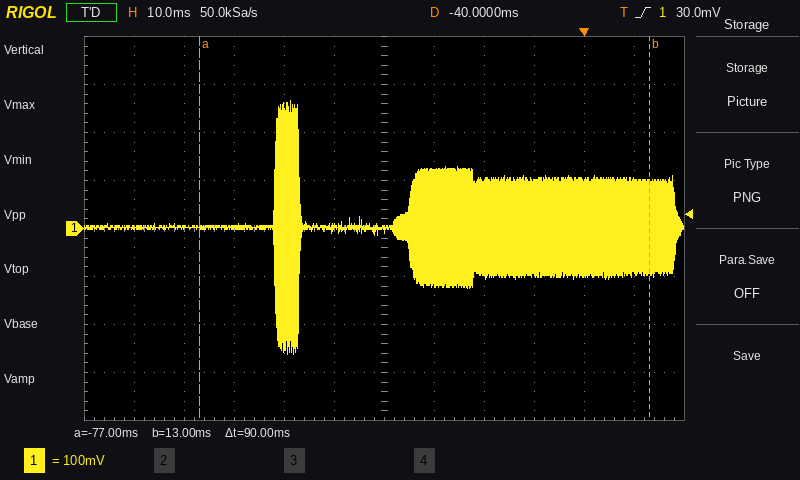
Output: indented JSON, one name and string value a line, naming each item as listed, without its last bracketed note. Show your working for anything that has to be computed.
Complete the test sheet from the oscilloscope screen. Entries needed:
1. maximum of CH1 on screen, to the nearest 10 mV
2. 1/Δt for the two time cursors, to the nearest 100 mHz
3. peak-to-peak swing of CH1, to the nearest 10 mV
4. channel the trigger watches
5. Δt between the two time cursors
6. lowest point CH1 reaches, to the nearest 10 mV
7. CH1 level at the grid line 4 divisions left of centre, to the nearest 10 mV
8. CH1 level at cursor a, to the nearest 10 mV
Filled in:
{
  "maximum of CH1 on screen, to the nearest 10 mV": "270 mV",
  "1/Δt for the two time cursors, to the nearest 100 mHz": "1 / 90 ms ≈ 11.1 Hz",
  "peak-to-peak swing of CH1, to the nearest 10 mV": "270 mV − (-260 mV) = 530 mV",
  "channel the trigger watches": "CH1",
  "Δt between the two time cursors": "90 ms",
  "lowest point CH1 reaches, to the nearest 10 mV": "-260 mV",
  "CH1 level at the grid line 4 divisions left of centre, to the nearest 10 mV": "0 mV",
  "CH1 level at cursor a, to the nearest 10 mV": "0 mV"
}
